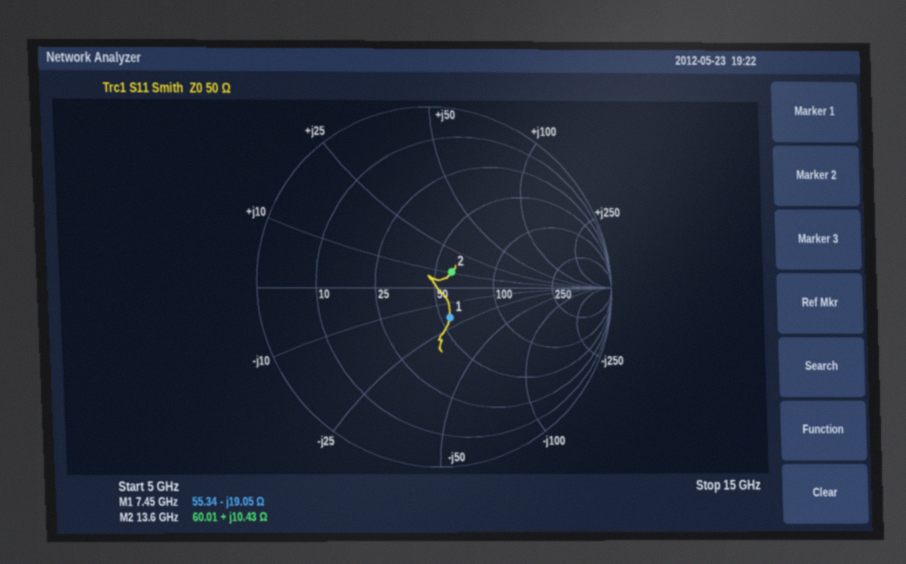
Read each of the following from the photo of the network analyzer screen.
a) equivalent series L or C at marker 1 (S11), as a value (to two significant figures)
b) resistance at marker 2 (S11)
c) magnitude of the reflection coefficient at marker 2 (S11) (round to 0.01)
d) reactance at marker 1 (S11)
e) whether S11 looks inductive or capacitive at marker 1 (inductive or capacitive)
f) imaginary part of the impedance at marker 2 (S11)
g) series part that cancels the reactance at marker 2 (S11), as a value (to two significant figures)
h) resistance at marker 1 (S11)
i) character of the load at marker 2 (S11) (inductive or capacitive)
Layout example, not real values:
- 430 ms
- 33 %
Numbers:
- 1.1 pF
- 60.01 Ω
- 0.13
- -19.05 Ω
- capacitive
- +10.43 Ω
- 1.1 pF
- 55.34 Ω
- inductive
